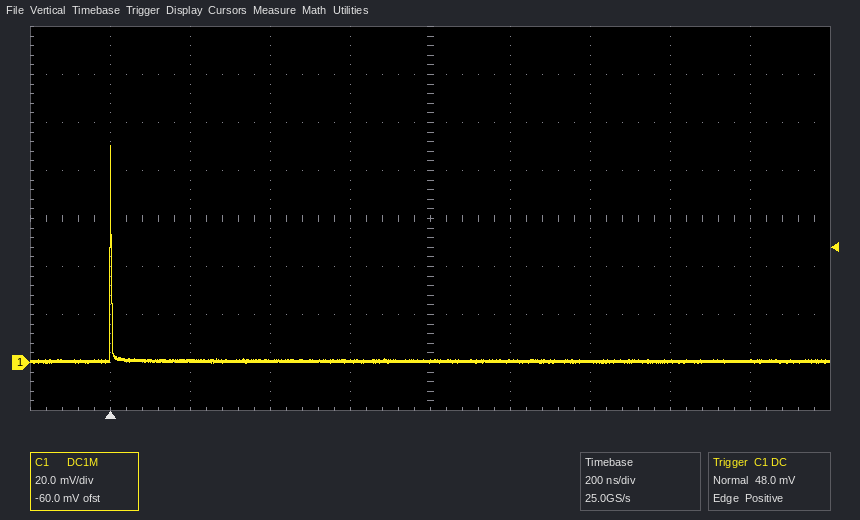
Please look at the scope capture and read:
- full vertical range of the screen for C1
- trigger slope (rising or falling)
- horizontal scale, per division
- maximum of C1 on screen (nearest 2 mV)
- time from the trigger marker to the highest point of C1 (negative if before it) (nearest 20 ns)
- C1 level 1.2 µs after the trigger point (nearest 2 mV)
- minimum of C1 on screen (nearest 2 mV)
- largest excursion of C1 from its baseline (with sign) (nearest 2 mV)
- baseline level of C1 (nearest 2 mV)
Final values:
160 mV
rising
200 ns
90 mV
0 ns
0 mV
0 mV
+90 mV
0 mV
